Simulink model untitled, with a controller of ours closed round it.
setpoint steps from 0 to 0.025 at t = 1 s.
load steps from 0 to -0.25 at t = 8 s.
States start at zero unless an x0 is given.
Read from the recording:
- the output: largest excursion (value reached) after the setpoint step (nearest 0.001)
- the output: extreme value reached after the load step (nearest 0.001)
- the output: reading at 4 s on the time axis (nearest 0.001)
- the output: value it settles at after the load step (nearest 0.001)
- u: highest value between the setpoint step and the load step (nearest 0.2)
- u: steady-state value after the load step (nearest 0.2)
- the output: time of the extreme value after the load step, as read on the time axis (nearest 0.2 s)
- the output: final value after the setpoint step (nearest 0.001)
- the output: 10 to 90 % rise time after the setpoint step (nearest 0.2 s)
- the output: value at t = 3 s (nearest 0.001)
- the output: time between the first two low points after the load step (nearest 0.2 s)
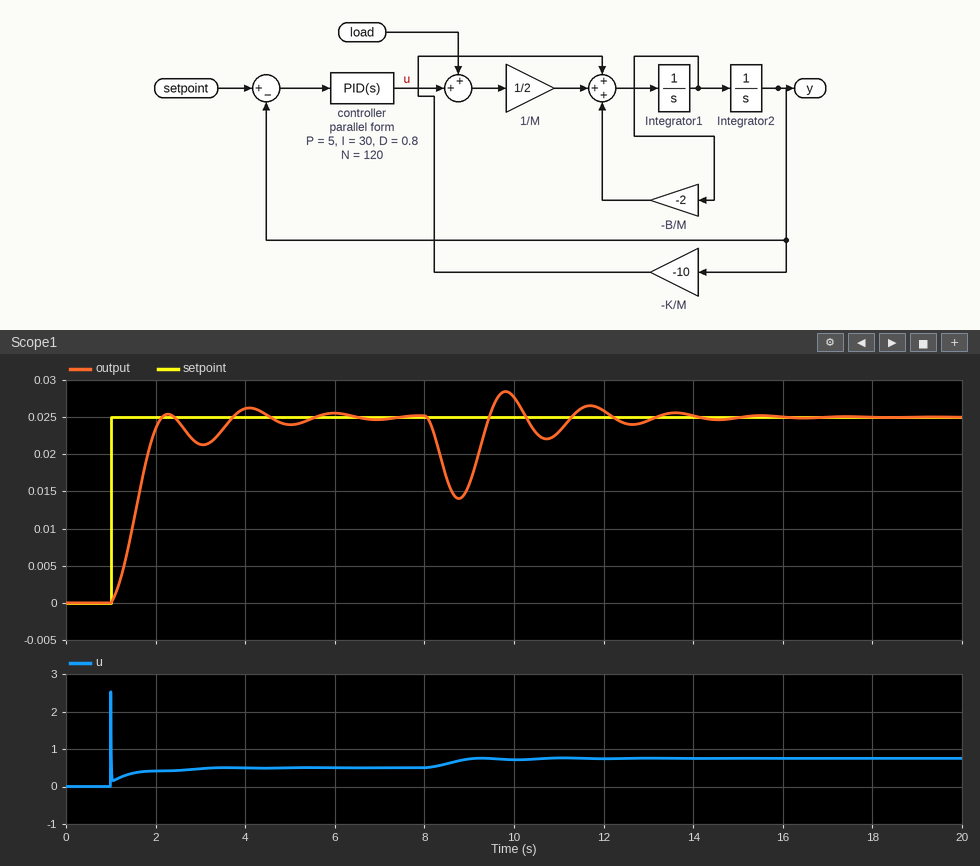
0.026
0.014
0.026
0.025
2.6
0.8
8.8 s
0.025
0.8 s
0.021
2.0 s
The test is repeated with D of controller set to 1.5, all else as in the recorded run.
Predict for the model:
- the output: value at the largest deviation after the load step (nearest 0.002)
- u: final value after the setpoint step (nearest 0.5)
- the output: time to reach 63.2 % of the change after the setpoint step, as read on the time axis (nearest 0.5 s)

0.014
0.5
1.5 s
